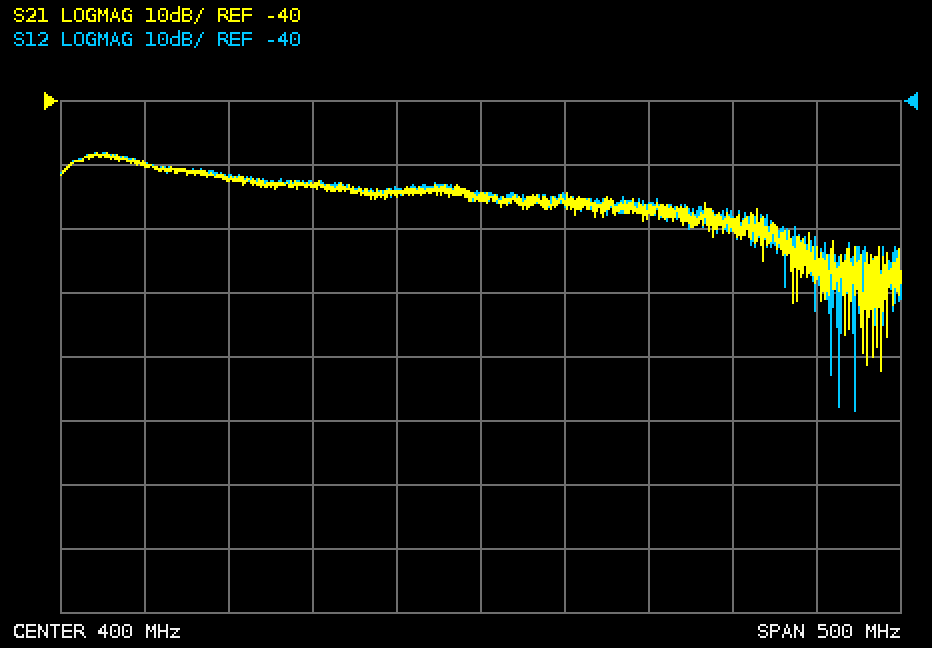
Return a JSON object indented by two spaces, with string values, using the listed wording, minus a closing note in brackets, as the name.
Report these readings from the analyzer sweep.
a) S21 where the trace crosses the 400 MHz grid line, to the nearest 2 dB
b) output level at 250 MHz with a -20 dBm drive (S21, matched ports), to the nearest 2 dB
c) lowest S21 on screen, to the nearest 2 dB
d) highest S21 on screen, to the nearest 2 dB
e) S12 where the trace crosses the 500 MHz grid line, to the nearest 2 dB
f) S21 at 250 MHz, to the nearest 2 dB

{
  "S21 where the trace crosses the 400 MHz grid line, to the nearest 2 dB": "-56 dB",
  "output level at 250 MHz with a -20 dBm drive (S21, matched ports), to the nearest 2 dB": "-72 dBm",
  "lowest S21 on screen, to the nearest 2 dB": "-82 dB",
  "highest S21 on screen, to the nearest 2 dB": "-48 dB",
  "S12 where the trace crosses the 500 MHz grid line, to the nearest 2 dB": "-56 dB",
  "S21 at 250 MHz, to the nearest 2 dB": "-52 dB"
}
